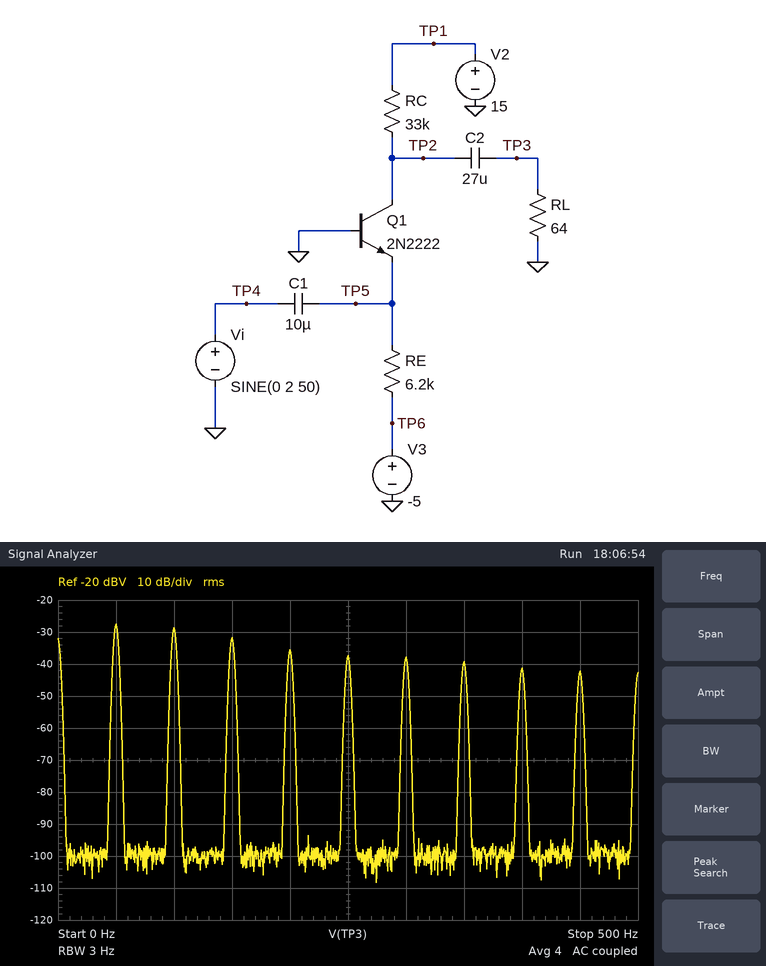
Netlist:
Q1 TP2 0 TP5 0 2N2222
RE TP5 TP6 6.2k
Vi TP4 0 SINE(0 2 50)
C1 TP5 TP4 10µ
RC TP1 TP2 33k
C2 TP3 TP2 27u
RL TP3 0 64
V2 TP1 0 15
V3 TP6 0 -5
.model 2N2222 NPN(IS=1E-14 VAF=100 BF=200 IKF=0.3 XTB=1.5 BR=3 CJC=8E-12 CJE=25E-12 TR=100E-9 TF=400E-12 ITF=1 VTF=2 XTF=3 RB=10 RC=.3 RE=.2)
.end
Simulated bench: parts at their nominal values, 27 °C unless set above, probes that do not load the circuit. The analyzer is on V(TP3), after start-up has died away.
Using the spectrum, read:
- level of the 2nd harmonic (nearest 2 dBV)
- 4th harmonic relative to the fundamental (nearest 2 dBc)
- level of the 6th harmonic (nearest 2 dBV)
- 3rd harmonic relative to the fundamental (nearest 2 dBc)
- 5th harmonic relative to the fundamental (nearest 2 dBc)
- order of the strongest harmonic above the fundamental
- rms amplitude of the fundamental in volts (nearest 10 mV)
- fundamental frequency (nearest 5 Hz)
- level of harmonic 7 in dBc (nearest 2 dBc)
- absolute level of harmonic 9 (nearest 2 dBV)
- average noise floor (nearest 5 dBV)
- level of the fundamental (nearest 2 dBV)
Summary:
-28 dBV
-8 dBc
-38 dBV
-4 dBc
-10 dBc
2
40 mV
50 Hz
-12 dBc
-42 dBV
-100 dBV
-28 dBV
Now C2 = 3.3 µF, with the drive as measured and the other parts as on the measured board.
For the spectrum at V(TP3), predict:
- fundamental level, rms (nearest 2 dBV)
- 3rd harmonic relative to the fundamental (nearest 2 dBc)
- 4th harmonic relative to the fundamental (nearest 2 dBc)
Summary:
-28 dBV
-2 dBc
-2 dBc
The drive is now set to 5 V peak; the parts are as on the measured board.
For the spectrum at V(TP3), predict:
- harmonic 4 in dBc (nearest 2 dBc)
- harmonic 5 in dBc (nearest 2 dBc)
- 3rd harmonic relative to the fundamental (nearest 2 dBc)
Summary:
-4 dBc
-8 dBc
-2 dBc
